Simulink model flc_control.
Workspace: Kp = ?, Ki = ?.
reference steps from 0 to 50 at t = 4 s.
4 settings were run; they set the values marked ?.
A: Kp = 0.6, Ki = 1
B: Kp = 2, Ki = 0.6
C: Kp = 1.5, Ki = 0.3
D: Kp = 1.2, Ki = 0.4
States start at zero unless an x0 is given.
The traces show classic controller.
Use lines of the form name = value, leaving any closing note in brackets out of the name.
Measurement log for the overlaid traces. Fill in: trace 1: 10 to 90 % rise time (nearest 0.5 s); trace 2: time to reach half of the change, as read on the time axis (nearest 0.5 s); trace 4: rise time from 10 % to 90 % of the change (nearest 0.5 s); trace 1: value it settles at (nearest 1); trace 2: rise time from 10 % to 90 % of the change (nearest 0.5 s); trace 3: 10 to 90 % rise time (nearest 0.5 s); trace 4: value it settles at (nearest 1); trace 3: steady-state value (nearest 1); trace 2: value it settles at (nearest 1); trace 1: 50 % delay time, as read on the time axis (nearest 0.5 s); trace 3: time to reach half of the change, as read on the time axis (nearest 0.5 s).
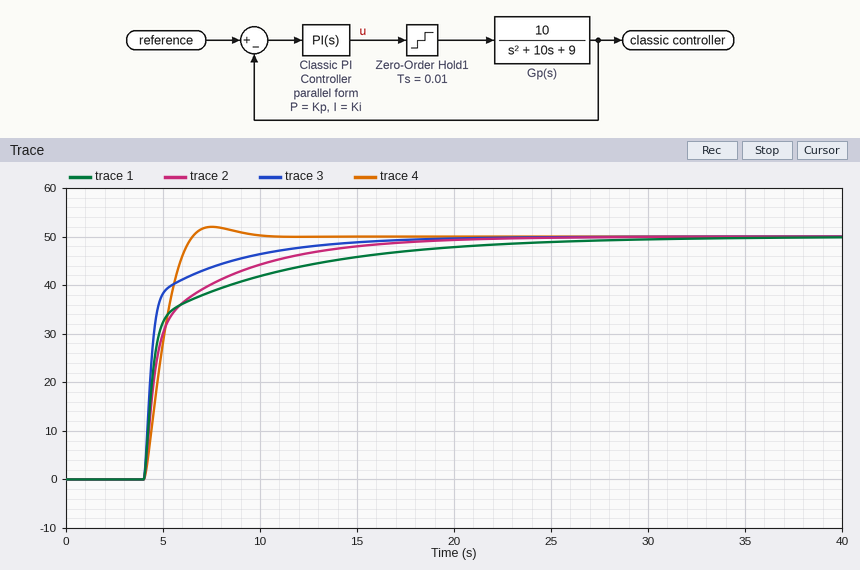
trace 1: 10 to 90 % rise time = 9.5 s
trace 2: time to reach half of the change, as read on the time axis = 4.5 s
trace 4: rise time from 10 % to 90 % of the change = 1.5 s
trace 1: value it settles at = 50
trace 2: rise time from 10 % to 90 % of the change = 6.5 s
trace 3: 10 to 90 % rise time = 4.5 s
trace 4: value it settles at = 50
trace 3: steady-state value = 50
trace 2: value it settles at = 50
trace 1: 50 % delay time, as read on the time axis = 4.5 s
trace 3: time to reach half of the change, as read on the time axis = 4.5 s
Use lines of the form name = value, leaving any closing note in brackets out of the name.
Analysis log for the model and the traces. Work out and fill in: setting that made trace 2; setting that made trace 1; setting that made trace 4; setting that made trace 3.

setting that made trace 2 = D
setting that made trace 1 = C
setting that made trace 4 = A
setting that made trace 3 = B
